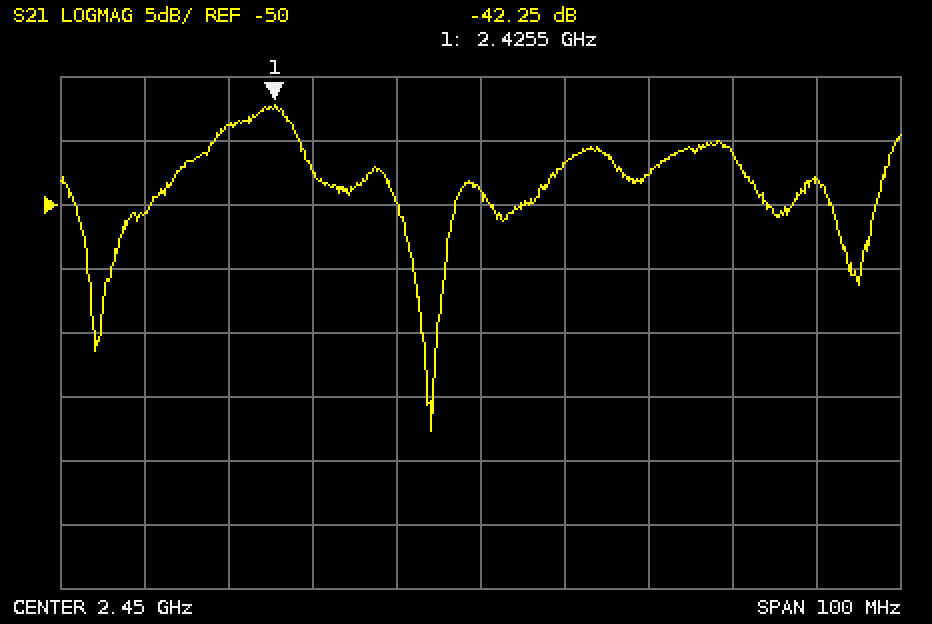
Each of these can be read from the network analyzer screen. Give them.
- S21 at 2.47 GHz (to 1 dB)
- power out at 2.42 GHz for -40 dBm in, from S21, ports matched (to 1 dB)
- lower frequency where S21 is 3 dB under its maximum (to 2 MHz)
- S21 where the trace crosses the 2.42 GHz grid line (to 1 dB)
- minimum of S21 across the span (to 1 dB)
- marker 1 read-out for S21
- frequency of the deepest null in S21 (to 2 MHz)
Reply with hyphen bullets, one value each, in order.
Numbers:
- -48 dB
- -84 dBm
- 2.418 GHz
- -44 dB
- -68 dB
- -42.25 dB
- 2.444 GHz
